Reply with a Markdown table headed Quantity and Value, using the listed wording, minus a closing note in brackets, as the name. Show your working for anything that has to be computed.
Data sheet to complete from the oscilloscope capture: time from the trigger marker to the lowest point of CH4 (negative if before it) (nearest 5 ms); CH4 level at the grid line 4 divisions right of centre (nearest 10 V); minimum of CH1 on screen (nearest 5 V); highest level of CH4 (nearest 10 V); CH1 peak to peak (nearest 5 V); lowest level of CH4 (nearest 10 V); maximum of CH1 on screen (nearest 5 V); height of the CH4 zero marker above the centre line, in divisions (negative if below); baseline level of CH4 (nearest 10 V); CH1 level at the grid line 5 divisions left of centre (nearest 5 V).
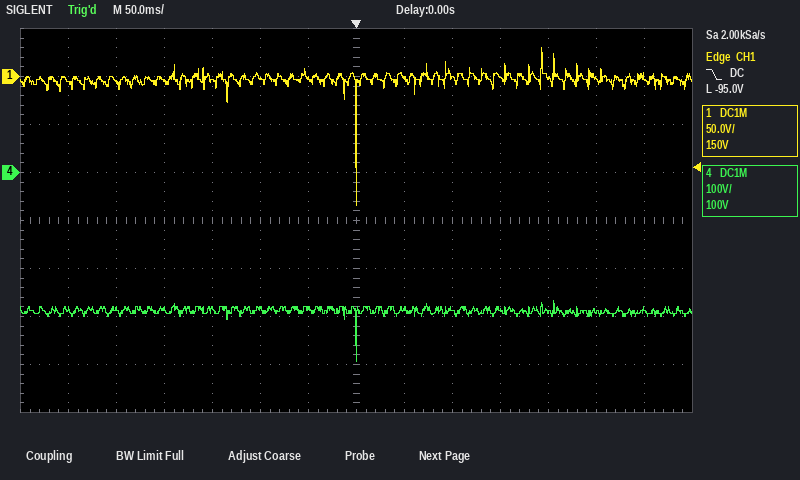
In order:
| Quantity | Value |
|---|---|
| time from the trigger marker to the lowest point of CH4 (negative if before it) | 0 ms |
| CH4 level at the grid line 4 divisions right of centre | -290 V |
| minimum of CH1 on screen | -135 V |
| highest level of CH4 | -270 V |
| CH1 peak to peak | 30 V − (-135 V) = 165 V |
| lowest level of CH4 | -390 V |
| maximum of CH1 on screen | 30 V |
| height of the CH4 zero marker above the centre line, in divisions | +1.0 div |
| baseline level of CH4 | -290 V |
| CH1 level at the grid line 5 divisions left of centre | -5 V |
